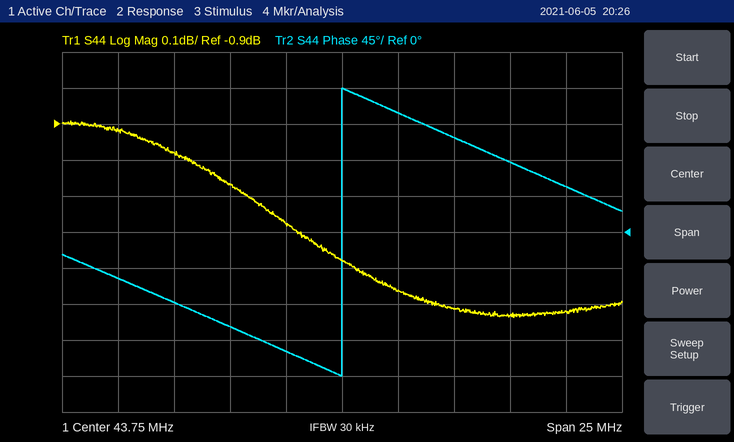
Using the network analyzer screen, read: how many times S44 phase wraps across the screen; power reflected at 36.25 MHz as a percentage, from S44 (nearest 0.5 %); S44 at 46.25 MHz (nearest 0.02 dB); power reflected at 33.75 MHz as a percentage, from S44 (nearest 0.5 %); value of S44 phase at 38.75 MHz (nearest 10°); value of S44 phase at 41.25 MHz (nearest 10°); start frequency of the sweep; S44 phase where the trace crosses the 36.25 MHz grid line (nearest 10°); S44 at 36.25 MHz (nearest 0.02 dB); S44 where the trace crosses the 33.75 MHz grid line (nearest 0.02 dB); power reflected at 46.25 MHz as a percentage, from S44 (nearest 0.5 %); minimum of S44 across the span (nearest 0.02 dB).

1
80.0 %
-1.36 dB
81.0 %
-120°
-150°
31.25 MHz
-90°
-0.98 dB
-0.92 dB
73.0 %
-1.44 dB
